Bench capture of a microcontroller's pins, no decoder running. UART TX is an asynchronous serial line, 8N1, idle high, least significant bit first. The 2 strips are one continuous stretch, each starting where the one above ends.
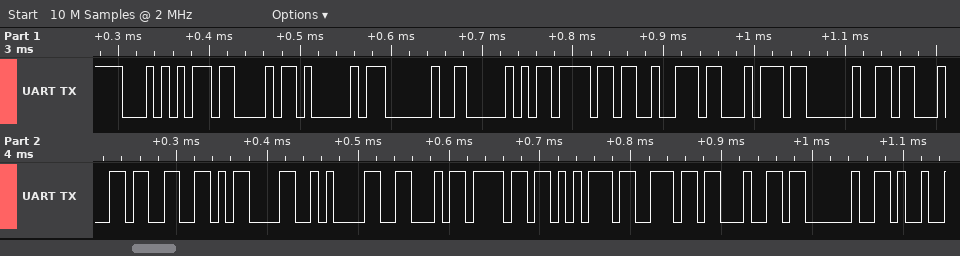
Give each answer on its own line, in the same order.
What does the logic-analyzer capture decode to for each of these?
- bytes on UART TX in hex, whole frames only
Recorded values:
54 43 41 20 50 6F 72 74 20 23 33 0D 0A 46 6F 75 6E 64 20
